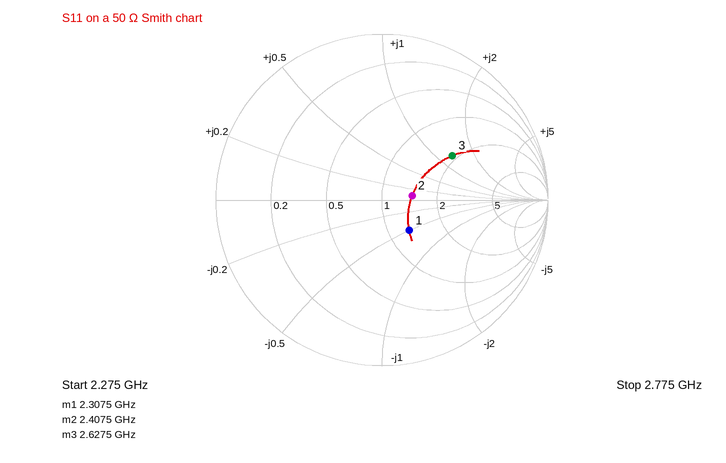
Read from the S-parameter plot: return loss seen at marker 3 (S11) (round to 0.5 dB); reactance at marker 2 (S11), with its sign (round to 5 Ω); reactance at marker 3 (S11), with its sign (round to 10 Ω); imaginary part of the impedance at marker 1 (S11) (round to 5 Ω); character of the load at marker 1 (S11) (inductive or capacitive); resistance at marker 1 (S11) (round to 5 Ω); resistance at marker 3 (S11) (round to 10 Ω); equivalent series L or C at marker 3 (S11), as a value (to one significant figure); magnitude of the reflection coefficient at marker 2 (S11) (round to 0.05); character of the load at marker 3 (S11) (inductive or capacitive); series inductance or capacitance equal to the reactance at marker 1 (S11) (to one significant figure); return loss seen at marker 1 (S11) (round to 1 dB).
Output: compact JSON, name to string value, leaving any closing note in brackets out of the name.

{"return loss seen at marker 3 (S11)": "6.0 dB", "reactance at marker 2 (S11), with its sign": "+5 Ω", "reactance at marker 3 (S11), with its sign": "+70 Ω", "imaginary part of the impedance at marker 1 (S11)": "-25 Ω", "character of the load at marker 1 (S11)": "capacitive", "resistance at marker 1 (S11)": "65 Ω", "resistance at marker 3 (S11)": "90 Ω", "equivalent series L or C at marker 3 (S11), as a value": "4 nH", "magnitude of the reflection coefficient at marker 2 (S11)": "0.20", "character of the load at marker 3 (S11)": "inductive", "series inductance or capacitance equal to the reactance at marker 1 (S11)": "3 pF", "return loss seen at marker 1 (S11)": "12 dB"}
